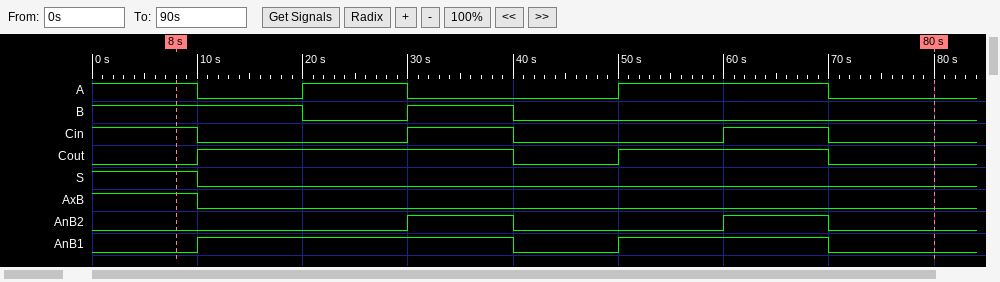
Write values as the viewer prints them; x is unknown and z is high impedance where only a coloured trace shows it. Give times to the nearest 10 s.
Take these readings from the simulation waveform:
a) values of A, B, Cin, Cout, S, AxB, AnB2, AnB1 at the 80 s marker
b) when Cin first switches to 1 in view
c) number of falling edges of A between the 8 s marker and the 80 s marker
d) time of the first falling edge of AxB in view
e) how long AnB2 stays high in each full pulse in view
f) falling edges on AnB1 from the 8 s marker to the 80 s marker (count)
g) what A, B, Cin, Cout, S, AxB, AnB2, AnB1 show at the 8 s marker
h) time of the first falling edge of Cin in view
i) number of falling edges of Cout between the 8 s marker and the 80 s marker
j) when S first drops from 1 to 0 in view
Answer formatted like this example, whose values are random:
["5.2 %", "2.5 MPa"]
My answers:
["A=0, B=0, Cin=0, Cout=0, S=0, AxB=0, AnB2=0, AnB1=0", "30 s", "3", "10 s", "10 s, 10 s", "2", "A=1, B=1, Cin=1, Cout=0, S=1, AxB=1, AnB2=0, AnB1=0", "10 s", "2", "10 s"]
